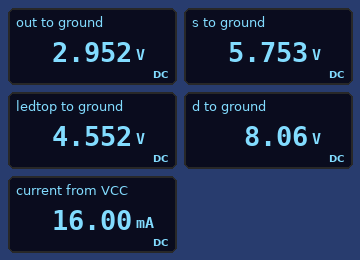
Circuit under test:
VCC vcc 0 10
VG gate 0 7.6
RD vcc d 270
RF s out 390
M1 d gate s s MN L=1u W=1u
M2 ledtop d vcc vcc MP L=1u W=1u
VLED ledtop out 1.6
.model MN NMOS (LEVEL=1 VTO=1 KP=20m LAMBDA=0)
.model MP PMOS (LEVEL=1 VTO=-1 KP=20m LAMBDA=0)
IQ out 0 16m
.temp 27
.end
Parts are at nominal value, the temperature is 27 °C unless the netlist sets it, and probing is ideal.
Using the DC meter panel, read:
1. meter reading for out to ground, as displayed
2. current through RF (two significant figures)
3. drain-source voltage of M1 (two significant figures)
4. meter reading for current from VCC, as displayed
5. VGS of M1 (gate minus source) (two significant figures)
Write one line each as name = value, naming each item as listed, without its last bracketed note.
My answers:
meter reading for out to ground, as displayed = 2.952 V
current through RF = 7.2 mA
drain-source voltage of M1 = 2.3 V
meter reading for current from VCC, as displayed = 16.00 mA
VGS of M1 (gate minus source) = 1.8 V
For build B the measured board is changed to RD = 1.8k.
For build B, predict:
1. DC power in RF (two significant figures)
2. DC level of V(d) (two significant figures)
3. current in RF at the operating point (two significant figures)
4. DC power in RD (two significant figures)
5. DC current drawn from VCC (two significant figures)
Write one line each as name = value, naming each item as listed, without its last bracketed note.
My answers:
DC power in RF = 590 µW
DC level of V(d) = 7.8 V
current in RF at the operating point = 1.2 mA
DC power in RD = 2.7 mW
DC current drawn from VCC = 16 mA
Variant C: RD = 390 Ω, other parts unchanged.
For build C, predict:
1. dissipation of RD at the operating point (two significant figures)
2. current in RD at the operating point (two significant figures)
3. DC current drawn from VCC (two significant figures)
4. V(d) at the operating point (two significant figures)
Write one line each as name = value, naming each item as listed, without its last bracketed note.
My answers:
dissipation of RD at the operating point = 11 mW
current in RD at the operating point = 5.2 mA
DC current drawn from VCC = 16 mA
V(d) at the operating point = 8.0 V
